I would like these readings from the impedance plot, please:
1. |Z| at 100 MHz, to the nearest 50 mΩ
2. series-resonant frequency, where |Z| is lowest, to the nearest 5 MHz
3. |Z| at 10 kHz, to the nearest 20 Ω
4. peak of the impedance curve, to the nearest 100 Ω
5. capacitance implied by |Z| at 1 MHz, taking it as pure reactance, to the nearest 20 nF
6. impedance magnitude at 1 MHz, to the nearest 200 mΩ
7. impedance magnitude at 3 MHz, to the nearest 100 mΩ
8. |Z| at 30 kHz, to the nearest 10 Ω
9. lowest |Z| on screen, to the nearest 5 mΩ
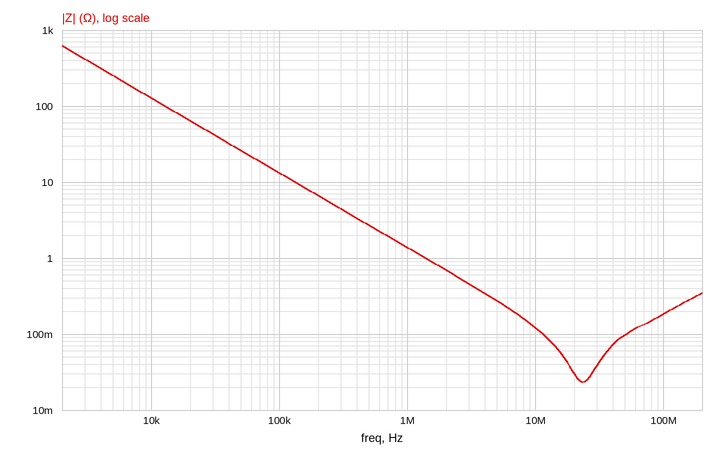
200 mΩ
25 MHz
120 Ω
600 Ω
120 nF
1.4 Ω
500 mΩ
40 Ω
25 mΩ
